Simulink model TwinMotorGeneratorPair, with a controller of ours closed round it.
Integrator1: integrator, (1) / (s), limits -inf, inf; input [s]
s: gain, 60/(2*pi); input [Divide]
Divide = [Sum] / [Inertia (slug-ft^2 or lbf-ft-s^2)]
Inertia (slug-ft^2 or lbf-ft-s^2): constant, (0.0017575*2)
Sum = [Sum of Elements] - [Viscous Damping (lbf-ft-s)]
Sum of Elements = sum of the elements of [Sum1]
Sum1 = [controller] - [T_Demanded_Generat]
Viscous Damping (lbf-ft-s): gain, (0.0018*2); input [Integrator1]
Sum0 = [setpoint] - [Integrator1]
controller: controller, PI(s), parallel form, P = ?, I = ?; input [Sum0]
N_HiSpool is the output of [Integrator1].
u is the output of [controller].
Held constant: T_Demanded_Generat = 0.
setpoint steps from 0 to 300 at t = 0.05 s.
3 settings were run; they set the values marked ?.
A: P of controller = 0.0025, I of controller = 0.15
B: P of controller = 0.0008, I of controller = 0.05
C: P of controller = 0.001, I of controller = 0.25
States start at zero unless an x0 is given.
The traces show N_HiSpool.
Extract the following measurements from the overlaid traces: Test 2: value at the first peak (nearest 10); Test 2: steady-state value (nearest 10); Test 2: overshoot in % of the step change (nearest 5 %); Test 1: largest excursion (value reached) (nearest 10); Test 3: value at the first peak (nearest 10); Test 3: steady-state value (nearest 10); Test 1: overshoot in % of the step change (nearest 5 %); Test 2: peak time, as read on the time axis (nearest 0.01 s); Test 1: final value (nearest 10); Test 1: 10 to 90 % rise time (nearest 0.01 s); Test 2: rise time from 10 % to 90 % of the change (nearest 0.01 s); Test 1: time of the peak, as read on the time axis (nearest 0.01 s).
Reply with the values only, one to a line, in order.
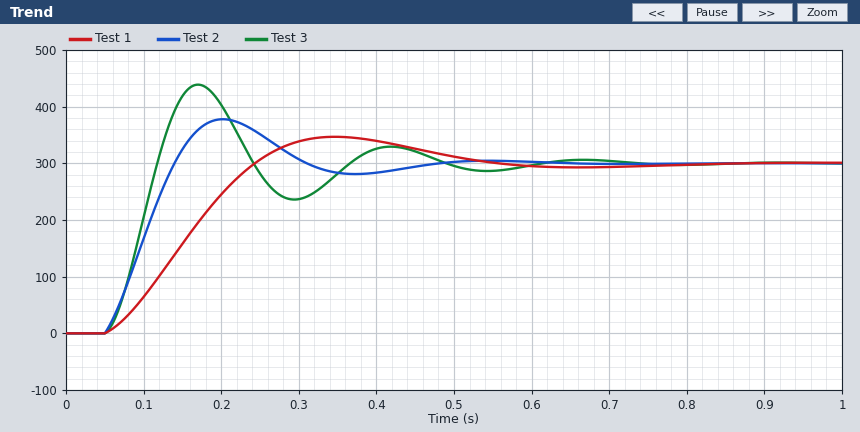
380
300
25 %
350
440
300
15 %
0.20 s
300
0.14 s
0.07 s
0.35 s
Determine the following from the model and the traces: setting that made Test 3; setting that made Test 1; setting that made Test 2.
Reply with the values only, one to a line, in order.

C
B
A
